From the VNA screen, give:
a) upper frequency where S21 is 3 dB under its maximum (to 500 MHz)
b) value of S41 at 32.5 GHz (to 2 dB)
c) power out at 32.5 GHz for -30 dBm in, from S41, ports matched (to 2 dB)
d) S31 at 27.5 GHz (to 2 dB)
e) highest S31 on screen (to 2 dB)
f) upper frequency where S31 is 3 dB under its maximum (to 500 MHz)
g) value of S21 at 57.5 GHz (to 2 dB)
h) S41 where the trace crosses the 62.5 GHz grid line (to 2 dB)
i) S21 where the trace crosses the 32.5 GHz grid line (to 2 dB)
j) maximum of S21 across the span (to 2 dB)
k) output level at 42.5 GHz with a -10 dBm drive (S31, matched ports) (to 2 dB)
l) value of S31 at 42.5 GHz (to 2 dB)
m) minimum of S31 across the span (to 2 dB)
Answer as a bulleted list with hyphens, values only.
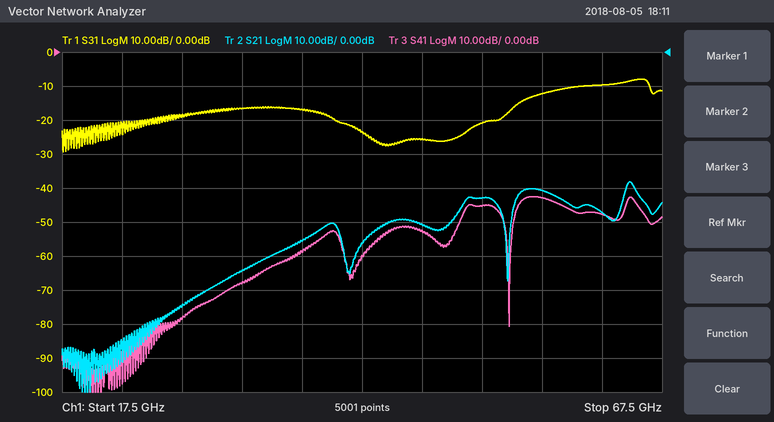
- 65.5 GHz
- -68 dB
- -98 dBm
- -18 dB
- -8 dB
- 66.5 GHz
- -40 dB
- -48 dB
- -64 dB
- -38 dB
- -34 dBm
- -24 dB
- -30 dB
